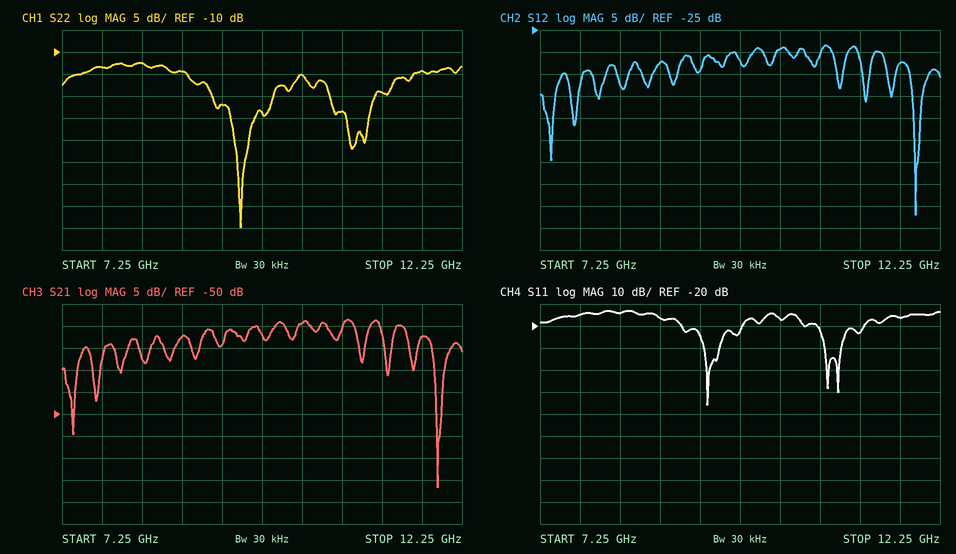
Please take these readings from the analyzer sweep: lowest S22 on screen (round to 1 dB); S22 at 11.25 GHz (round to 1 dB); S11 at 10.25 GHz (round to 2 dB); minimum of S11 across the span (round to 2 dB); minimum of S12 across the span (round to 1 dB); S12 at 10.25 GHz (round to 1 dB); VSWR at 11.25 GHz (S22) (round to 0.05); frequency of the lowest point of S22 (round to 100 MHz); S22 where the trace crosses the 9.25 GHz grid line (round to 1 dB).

-50 dB
-19 dB
-16 dB
-56 dB
-67 dB
-29 dB
1.25
9.5 GHz
-22 dB
